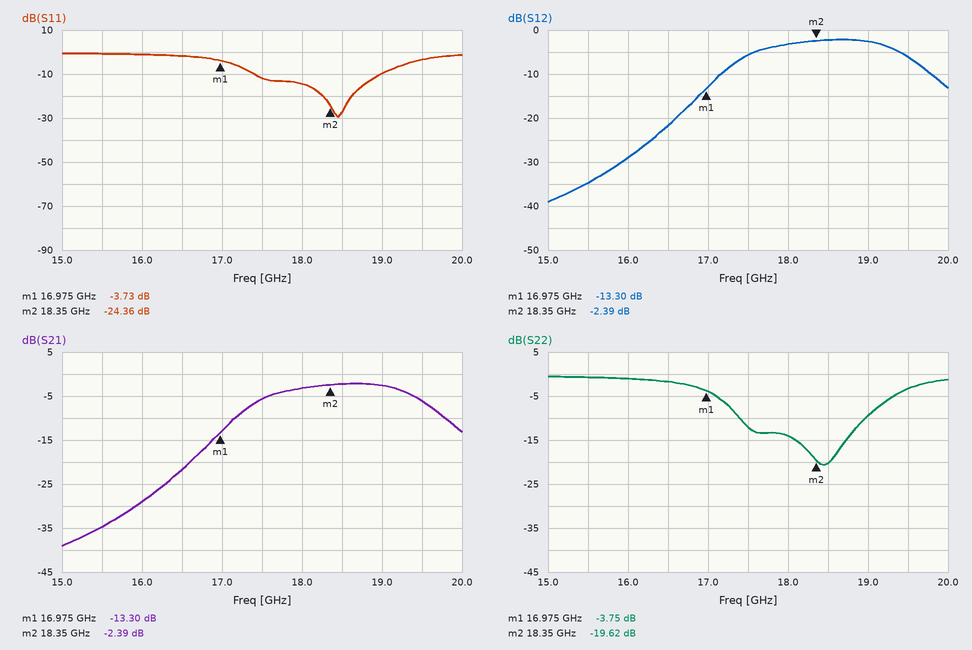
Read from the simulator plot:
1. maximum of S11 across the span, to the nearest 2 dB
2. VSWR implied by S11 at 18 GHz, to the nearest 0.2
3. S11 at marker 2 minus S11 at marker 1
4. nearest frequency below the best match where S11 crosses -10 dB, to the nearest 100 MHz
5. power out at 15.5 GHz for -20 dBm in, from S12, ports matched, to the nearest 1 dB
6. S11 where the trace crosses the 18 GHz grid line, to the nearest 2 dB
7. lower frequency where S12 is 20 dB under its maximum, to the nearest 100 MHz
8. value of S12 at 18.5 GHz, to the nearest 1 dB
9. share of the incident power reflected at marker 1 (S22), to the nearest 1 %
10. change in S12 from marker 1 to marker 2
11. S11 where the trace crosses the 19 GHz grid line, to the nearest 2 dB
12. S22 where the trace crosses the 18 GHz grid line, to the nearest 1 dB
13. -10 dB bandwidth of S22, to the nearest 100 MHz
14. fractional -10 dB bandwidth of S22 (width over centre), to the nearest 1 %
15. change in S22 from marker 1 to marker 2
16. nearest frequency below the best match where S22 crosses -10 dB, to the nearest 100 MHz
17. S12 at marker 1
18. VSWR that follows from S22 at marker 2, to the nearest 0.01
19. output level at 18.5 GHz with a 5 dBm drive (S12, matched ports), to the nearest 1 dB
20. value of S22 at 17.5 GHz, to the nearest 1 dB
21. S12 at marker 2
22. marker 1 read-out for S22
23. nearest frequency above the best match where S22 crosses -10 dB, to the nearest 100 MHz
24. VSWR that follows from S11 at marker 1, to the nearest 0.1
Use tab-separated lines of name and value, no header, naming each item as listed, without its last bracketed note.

maximum of S11 across the span, to the nearest 2 dB	0 dB
VSWR implied by S11 at 18 GHz, to the nearest 0.2	1.4
S11 at marker 2 minus S11 at marker 1	-20.63 dB
nearest frequency below the best match where S11 crosses -10 dB, to the nearest 100 MHz	17.4 GHz
power out at 15.5 GHz for -20 dBm in, from S12, ports matched, to the nearest 1 dB	-55 dBm
S11 where the trace crosses the 18 GHz grid line, to the nearest 2 dB	-14 dB
lower frequency where S12 is 20 dB under its maximum, to the nearest 100 MHz	16.5 GHz
value of S12 at 18.5 GHz, to the nearest 1 dB	-2 dB
share of the incident power reflected at marker 1 (S22), to the nearest 1 %	42 %
change in S12 from marker 1 to marker 2	10.91 dB
S11 where the trace crosses the 19 GHz grid line, to the nearest 2 dB	-10 dB
S22 where the trace crosses the 18 GHz grid line, to the nearest 1 dB	-14 dB
-10 dB bandwidth of S22, to the nearest 100 MHz	1.6 GHz
fractional -10 dB bandwidth of S22 (width over centre), to the nearest 1 %	9 %
change in S22 from marker 1 to marker 2	-15.87 dB
nearest frequency below the best match where S22 crosses -10 dB, to the nearest 100 MHz	17.4 GHz
S12 at marker 1	-13.30 dB
VSWR that follows from S22 at marker 2, to the nearest 0.01	1.23
output level at 18.5 GHz with a 5 dBm drive (S12, matched ports), to the nearest 1 dB	3 dBm
value of S22 at 17.5 GHz, to the nearest 1 dB	-12 dB
S12 at marker 2	-2.39 dB
marker 1 read-out for S22	-3.75 dB
nearest frequency above the best match where S22 crosses -10 dB, to the nearest 100 MHz	19.0 GHz
VSWR that follows from S11 at marker 1, to the nearest 0.1	4.7
